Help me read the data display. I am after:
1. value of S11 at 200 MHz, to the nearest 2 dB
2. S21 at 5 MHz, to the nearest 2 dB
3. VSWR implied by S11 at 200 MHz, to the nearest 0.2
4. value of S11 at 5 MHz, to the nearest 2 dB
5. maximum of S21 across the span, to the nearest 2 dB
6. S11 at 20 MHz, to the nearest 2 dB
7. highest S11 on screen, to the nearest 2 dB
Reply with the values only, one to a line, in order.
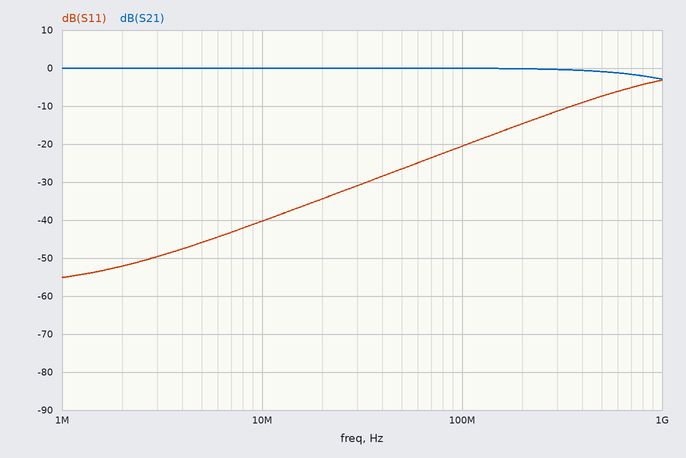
-14 dB
0 dB
1.4
-46 dB
0 dB
-34 dB
-4 dB
